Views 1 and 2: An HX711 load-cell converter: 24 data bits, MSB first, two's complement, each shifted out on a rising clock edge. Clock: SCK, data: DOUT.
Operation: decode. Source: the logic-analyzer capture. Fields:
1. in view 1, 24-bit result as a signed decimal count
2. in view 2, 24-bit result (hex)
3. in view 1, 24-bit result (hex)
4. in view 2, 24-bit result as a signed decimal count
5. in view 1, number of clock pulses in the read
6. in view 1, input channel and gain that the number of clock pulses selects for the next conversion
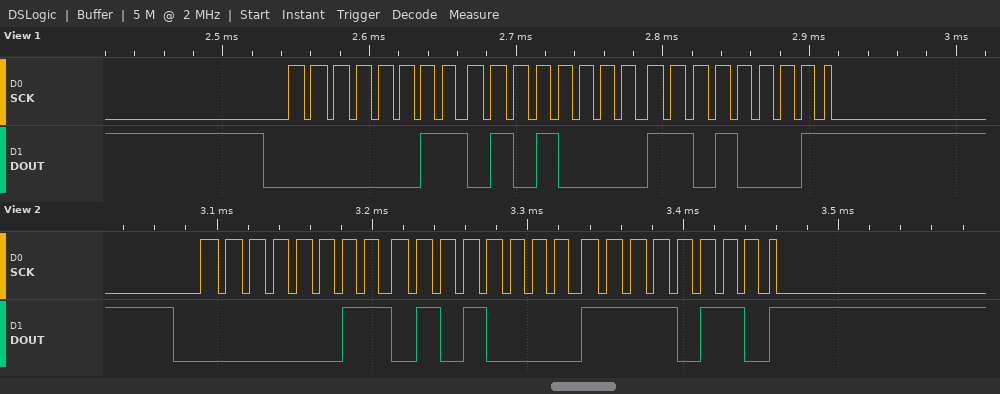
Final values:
217297
0x0350F6
0x0350D1
217334
25
channel A, gain 128
